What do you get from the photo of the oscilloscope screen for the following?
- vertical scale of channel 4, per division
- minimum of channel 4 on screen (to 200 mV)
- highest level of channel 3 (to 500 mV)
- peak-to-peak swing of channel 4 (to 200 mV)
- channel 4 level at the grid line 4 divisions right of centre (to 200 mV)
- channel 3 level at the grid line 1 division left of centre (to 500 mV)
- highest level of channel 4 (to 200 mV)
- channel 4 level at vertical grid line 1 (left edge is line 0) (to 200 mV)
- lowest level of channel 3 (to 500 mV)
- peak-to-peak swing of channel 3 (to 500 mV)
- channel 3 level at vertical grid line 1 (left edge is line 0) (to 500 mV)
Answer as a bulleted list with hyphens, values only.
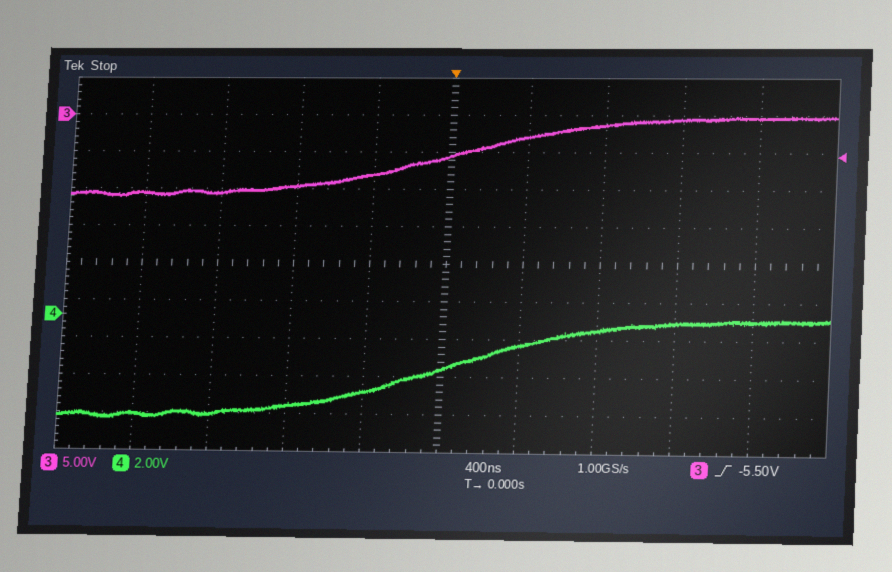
- 2 V
- -5.4 V
- 0.0 V
- 5.4 V
- -200 mV
- -8.0 V
- 0.0 V
- -5.2 V
- -11.0 V
- 11.0 V
- -10.5 V
